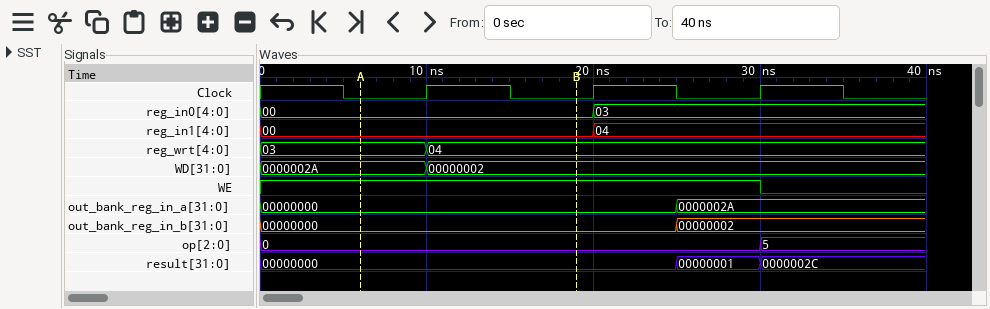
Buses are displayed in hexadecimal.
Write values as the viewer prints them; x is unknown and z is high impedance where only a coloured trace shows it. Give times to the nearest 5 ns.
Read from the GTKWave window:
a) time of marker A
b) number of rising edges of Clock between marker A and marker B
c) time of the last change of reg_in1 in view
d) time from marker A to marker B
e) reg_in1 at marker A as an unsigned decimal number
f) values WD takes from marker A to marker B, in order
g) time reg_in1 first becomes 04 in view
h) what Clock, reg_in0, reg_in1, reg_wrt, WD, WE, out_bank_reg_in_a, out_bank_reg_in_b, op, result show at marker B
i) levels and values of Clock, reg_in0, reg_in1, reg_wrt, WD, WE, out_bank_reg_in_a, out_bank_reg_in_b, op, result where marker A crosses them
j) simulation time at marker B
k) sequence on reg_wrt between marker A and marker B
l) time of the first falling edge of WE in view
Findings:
5 ns
1
20 ns
15 ns
0
0000002A, 00000002
20 ns
Clock=0, reg_in0=00, reg_in1=00, reg_wrt=04, WD=00000002, WE=1, out_bank_reg_in_a=00000000, out_bank_reg_in_b=00000000, op=0, result=00000000
Clock=0, reg_in0=00, reg_in1=00, reg_wrt=03, WD=0000002A, WE=1, out_bank_reg_in_a=00000000, out_bank_reg_in_b=00000000, op=0, result=00000000
20 ns
03, 04
30 ns
